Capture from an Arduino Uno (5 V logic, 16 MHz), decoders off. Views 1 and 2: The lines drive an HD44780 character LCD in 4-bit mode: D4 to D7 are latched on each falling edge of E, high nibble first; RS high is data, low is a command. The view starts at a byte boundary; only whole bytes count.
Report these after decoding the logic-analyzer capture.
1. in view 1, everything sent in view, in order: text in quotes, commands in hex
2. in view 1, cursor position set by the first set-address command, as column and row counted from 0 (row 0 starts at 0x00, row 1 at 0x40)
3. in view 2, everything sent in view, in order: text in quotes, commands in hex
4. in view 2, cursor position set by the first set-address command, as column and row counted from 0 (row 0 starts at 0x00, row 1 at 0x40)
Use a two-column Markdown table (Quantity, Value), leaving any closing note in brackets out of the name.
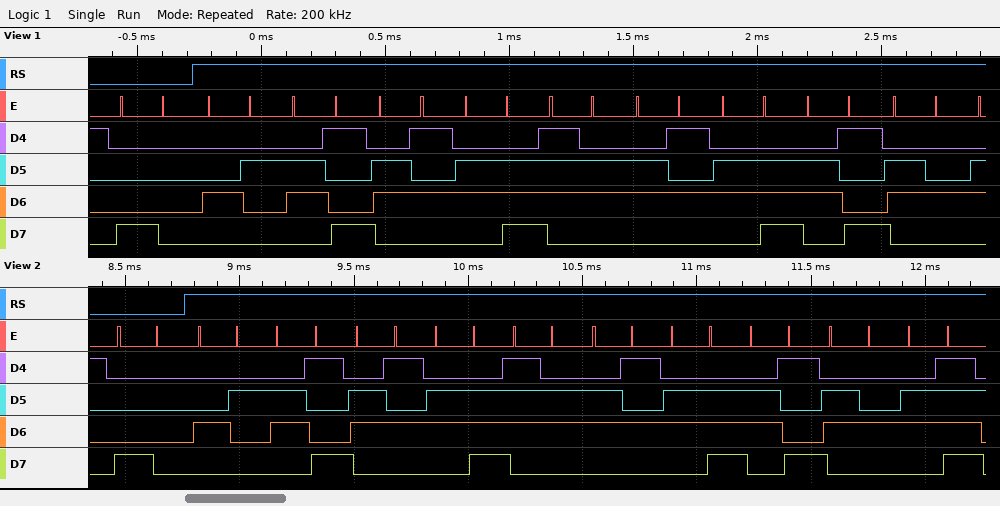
| Quantity | Value |
|---|---|
| in view 1, everything sent in view, in order: text in quotes, commands in hex | 0x80 "Bienvenid" |
| in view 1, cursor position set by the first set-address command, as column and row counted from 0 | column 0, row 0 |
| in view 2, everything sent in view, in order: text in quotes, commands in hex | 0x80 "Bienvenido" |
| in view 2, cursor position set by the first set-address command, as column and row counted from 0 | column 0, row 0 |
